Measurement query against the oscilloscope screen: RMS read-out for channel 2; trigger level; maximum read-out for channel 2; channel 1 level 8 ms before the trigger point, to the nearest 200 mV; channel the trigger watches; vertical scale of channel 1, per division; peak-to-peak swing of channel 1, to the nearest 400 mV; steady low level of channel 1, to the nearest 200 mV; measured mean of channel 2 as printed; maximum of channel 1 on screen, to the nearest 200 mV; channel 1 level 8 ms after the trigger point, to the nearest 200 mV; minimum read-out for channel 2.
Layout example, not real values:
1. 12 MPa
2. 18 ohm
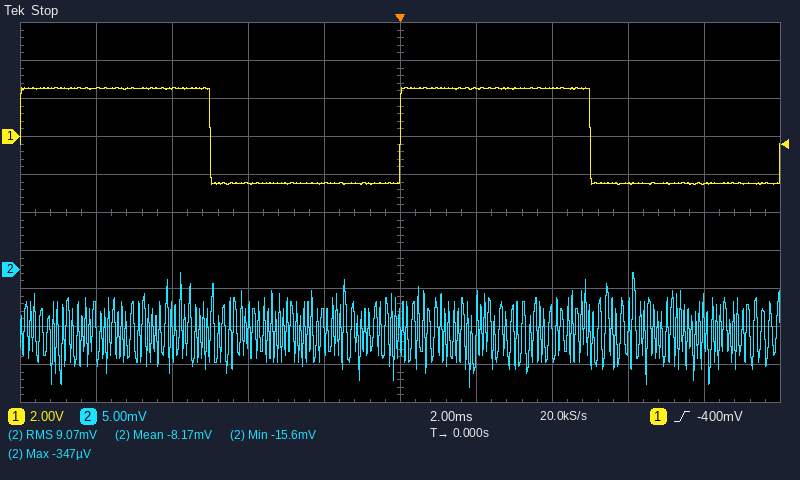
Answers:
1. 9.07 mV
2. -400 mV
3. -347 µV
4. 2.6 V
5. channel 1
6. 2 V
7. 5.2 V
8. -2.4 V
9. -8.17 mV
10. 2.6 V
11. -2.4 V
12. -15.6 mV
